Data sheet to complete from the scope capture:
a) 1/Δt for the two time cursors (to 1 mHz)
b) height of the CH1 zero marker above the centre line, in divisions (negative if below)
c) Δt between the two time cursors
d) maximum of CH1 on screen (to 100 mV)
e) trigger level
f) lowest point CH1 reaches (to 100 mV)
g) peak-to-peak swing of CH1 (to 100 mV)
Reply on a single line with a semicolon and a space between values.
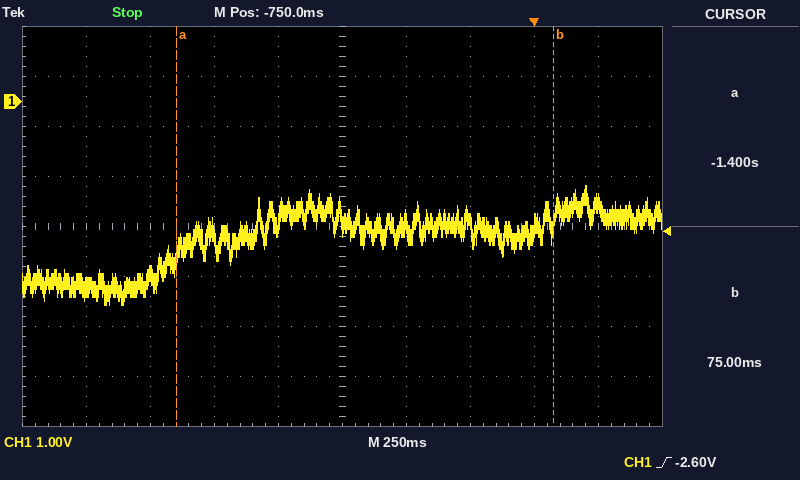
678 mHz; +2.5 div; 1.475 s; -1.7 V; -2.60 V; -4.1 V; 2.4 V
